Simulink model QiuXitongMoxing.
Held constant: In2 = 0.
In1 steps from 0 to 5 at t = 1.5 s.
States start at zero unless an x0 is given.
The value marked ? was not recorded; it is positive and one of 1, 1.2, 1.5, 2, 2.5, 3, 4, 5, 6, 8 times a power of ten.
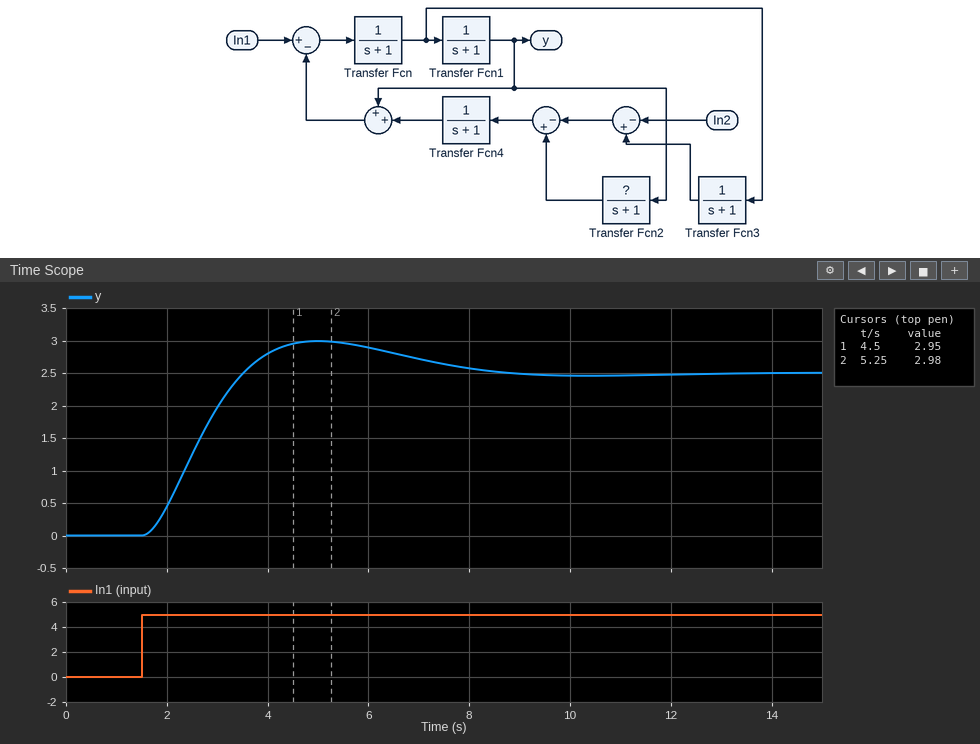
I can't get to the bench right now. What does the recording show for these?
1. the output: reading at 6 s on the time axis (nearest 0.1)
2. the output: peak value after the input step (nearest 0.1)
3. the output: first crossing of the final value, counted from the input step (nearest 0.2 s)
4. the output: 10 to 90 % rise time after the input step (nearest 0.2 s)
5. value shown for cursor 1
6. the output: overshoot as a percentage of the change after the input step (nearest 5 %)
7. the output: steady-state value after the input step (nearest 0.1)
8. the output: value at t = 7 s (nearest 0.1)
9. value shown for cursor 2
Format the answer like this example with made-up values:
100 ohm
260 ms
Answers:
2.9
3.0
2.0 s
1.4 s
2.95
20 %
2.5
2.7
2.98
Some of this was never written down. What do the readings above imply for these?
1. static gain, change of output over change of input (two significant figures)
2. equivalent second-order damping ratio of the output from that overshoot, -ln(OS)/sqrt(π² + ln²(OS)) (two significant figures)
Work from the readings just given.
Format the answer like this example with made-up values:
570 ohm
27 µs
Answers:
0.50
0.46
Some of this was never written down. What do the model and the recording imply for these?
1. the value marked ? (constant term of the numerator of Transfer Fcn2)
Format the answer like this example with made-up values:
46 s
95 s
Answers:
1
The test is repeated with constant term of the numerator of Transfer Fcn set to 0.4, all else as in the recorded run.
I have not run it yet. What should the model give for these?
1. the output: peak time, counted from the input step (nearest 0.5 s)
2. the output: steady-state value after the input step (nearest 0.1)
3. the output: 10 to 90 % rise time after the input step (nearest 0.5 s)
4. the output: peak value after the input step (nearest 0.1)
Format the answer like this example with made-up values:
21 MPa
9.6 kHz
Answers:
4.5 s
1.4
2.0 s
1.5
